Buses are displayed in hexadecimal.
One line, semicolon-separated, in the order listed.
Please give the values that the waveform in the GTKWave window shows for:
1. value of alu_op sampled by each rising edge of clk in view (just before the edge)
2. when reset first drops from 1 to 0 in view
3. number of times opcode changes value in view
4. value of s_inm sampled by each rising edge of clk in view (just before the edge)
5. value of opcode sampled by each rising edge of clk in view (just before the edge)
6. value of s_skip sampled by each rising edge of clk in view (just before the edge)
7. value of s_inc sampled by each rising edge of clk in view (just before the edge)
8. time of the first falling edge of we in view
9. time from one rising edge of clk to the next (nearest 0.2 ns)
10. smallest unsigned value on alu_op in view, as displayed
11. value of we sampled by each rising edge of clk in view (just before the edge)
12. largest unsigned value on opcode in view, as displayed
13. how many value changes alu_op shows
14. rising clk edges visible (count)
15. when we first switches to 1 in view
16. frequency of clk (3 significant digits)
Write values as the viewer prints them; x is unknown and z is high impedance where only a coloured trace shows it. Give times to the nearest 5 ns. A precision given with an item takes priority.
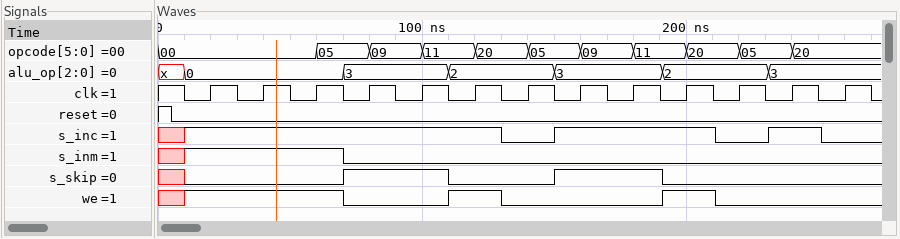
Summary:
0, 0, 0, 3, 3, 2, 2, 3, 3, 2, 2, 3, 3; 5 ns; 10; 1 1 1 0 0 0 0 0 0 0 0 0 0; 00, 00, 00, 05, 09, 11, 20, 05, 09, 11, 20, 05, 20; 0 0 0 1 1 0 0 1 1 0 0 0 0; 1 1 1 1 1 1 0 1 1 1 0 1 0; 70 ns; 20 ns; 0; 1 1 1 0 0 1 0 0 0 1 0 0 0; 20; 6; 13; 10 ns; 50.0 MHz
